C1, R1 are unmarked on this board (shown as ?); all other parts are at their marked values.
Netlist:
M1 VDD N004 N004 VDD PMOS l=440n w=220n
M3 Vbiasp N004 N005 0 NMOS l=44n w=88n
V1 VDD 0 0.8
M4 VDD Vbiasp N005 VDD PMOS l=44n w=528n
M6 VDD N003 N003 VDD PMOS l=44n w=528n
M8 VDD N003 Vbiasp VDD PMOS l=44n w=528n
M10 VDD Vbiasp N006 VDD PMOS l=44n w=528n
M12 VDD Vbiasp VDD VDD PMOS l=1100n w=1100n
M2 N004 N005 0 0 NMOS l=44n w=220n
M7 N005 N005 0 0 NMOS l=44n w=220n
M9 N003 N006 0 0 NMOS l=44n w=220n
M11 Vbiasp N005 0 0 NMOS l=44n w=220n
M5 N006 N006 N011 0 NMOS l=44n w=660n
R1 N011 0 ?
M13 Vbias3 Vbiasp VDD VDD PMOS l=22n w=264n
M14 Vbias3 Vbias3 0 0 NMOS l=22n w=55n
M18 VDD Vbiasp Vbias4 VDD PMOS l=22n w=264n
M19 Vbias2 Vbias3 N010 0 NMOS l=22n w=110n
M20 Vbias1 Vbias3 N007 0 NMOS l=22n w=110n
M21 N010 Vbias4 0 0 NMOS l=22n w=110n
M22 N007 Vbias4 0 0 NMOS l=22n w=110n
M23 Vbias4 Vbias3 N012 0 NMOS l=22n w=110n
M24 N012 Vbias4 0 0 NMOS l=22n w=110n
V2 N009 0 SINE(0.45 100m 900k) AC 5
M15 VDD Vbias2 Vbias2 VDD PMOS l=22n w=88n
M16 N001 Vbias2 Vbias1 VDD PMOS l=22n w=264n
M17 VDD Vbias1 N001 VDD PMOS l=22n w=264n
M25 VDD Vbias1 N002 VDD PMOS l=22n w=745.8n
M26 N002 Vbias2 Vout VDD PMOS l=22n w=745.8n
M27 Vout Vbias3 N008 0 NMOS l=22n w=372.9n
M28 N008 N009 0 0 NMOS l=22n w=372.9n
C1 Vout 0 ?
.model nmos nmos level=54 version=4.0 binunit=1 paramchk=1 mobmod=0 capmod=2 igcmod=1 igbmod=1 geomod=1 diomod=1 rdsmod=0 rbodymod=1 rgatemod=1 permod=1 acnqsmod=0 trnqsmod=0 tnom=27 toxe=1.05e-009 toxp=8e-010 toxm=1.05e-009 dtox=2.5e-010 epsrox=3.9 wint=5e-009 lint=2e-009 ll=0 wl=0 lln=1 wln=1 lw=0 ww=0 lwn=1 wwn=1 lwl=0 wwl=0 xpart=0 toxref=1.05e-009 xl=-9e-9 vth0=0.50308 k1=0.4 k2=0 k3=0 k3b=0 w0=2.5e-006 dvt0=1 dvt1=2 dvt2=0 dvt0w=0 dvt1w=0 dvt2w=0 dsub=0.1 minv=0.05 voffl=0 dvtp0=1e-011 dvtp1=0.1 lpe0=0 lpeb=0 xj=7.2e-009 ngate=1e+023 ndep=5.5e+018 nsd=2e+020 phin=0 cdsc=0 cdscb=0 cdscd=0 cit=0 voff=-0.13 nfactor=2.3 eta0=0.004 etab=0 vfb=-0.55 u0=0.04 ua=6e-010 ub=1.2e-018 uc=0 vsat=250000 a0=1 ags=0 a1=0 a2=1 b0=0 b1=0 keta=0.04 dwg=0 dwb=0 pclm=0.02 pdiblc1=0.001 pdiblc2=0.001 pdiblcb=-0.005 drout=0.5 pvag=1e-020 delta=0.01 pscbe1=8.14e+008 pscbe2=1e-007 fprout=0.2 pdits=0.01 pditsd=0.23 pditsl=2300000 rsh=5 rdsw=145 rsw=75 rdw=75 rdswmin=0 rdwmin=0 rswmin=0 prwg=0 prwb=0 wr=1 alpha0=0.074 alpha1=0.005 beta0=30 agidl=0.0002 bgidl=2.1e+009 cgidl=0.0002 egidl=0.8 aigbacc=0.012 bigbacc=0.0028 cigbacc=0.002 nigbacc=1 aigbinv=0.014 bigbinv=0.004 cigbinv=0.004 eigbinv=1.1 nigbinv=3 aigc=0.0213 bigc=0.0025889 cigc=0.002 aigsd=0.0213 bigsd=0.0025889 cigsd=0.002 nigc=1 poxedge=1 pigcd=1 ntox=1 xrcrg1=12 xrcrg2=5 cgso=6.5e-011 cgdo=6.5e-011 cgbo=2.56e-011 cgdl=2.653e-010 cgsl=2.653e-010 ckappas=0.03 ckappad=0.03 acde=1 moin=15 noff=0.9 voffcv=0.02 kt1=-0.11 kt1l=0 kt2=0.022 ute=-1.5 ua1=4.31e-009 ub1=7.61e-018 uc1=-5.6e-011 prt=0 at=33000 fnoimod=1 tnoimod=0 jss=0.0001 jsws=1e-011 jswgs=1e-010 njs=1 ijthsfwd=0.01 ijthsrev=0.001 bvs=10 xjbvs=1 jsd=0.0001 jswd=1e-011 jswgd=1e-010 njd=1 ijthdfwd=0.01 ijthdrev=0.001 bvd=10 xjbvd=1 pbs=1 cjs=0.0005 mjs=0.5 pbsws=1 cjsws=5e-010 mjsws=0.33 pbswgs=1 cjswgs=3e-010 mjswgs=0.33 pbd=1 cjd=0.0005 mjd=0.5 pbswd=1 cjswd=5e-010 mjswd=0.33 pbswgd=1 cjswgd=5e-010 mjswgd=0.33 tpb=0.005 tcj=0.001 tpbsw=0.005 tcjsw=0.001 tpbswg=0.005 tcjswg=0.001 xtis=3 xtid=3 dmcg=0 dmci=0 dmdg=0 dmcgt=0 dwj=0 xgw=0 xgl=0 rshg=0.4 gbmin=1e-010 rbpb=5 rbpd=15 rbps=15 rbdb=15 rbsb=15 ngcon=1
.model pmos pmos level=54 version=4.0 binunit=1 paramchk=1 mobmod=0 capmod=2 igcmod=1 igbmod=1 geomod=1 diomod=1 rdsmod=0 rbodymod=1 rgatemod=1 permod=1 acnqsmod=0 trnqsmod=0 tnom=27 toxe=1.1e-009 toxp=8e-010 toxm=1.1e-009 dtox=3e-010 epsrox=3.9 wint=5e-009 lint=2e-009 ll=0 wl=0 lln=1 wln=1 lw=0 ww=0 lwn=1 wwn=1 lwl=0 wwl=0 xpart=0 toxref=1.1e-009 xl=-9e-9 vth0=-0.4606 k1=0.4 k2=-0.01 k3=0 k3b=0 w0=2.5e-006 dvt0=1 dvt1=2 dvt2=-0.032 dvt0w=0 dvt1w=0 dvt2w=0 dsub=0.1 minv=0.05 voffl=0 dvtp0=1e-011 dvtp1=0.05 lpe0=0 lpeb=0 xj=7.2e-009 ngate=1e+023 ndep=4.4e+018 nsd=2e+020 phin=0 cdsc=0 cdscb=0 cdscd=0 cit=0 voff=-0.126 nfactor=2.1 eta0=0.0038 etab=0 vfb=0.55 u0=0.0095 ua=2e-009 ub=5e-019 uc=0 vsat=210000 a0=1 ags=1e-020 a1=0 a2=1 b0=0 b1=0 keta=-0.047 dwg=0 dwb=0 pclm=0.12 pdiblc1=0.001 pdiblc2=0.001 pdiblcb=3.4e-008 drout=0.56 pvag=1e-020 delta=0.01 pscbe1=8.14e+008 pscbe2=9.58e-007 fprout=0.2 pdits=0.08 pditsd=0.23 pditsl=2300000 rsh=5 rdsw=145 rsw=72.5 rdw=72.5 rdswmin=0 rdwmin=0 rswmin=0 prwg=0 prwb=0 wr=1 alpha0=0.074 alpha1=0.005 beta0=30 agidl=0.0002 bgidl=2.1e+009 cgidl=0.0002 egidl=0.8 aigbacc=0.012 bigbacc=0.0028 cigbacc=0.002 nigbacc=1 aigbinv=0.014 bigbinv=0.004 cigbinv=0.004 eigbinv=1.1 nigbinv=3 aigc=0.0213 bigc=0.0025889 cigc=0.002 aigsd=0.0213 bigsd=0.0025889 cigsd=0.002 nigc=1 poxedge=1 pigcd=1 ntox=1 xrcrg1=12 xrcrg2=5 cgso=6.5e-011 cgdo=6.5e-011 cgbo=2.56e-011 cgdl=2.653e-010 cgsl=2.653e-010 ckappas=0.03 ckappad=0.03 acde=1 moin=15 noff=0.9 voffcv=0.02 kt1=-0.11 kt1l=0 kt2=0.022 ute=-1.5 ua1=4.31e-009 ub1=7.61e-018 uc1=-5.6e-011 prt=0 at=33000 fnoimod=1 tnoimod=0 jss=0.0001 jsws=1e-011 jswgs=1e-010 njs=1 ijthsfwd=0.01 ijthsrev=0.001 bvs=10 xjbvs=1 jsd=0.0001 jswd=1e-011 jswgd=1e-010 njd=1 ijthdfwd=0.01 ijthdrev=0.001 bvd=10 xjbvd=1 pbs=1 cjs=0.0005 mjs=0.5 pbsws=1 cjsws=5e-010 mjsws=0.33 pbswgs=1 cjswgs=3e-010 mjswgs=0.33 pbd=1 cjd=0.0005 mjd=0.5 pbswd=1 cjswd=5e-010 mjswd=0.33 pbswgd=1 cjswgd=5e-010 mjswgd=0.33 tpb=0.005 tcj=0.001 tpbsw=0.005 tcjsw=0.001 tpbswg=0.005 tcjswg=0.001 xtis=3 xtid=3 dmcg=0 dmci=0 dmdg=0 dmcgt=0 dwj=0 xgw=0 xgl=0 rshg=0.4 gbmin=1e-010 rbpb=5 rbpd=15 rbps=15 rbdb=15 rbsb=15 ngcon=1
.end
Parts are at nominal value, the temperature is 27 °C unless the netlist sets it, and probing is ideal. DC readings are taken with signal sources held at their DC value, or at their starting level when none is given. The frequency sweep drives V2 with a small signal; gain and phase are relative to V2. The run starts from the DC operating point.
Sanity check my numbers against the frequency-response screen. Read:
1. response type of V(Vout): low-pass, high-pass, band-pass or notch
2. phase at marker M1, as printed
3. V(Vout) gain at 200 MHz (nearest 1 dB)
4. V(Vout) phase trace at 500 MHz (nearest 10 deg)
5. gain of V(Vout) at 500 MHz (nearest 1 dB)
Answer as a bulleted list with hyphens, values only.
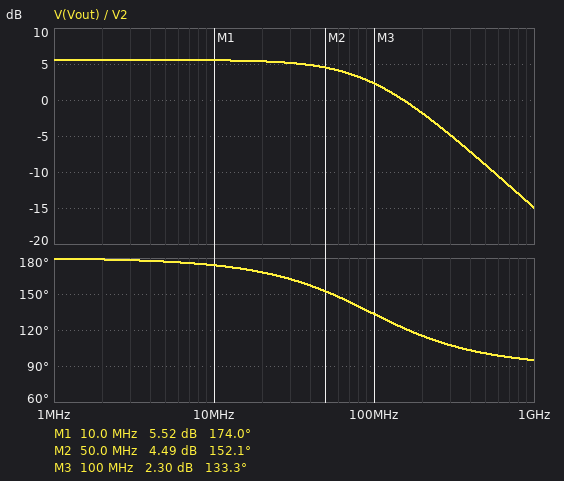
- low-pass
- 174.0 deg
- -2 dB
- 100 deg
- -9 dB
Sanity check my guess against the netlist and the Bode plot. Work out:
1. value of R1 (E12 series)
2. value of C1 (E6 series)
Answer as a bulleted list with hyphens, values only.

- 2.7 kΩ
- 330 fF
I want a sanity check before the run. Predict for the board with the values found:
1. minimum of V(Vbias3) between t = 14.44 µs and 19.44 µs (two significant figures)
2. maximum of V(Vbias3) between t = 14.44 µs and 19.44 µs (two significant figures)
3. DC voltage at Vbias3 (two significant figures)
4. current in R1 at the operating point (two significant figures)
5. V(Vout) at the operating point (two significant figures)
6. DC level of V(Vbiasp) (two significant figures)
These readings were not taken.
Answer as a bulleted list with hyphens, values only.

- 660 mV
- 660 mV
- 660 mV
- 24 µA
- 690 mV
- 160 mV
